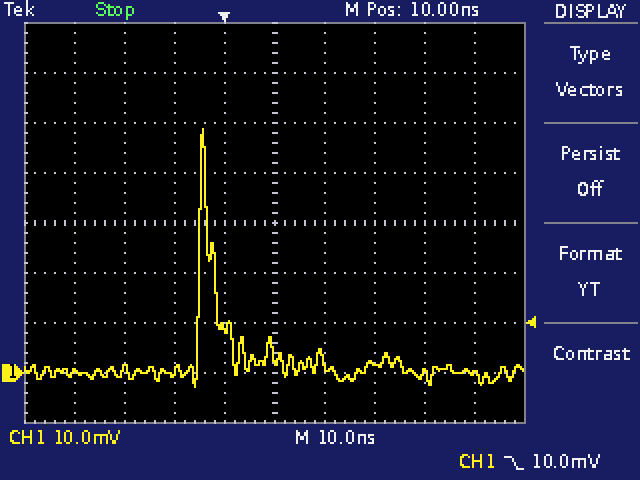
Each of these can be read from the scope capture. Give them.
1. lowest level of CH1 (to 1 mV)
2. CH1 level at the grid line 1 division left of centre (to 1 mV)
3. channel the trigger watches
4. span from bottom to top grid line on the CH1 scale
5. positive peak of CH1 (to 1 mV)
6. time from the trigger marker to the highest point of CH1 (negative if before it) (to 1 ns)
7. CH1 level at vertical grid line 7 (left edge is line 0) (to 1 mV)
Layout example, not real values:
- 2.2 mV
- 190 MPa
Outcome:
- -3 mV
- 9 mV
- CH1
- 80 mV
- 49 mV
- -4 ns
- 2 mV
